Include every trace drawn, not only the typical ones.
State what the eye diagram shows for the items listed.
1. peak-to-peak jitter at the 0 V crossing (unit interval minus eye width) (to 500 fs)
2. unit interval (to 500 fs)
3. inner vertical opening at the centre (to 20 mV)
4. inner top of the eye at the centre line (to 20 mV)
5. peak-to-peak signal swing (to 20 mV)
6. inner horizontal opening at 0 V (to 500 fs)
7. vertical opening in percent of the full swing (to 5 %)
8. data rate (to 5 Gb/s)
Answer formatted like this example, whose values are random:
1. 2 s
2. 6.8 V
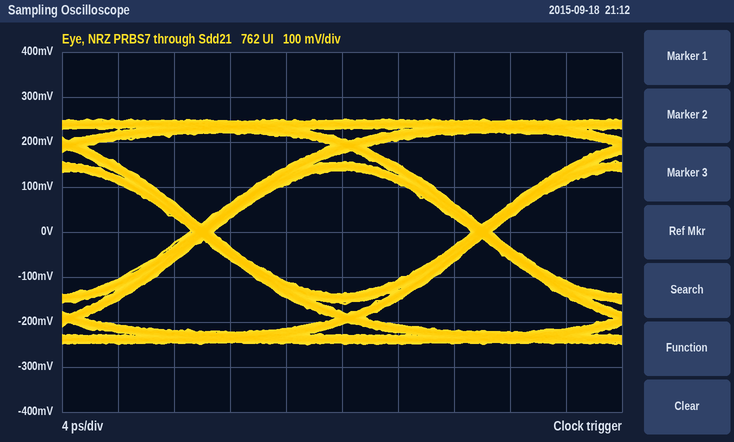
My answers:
1. 1.5 ps
2. 20.0 ps
3. 280 mV
4. 140 mV
5. 500 mV
6. 18.5 ps
7. 55 %
8. 50 Gb/s
